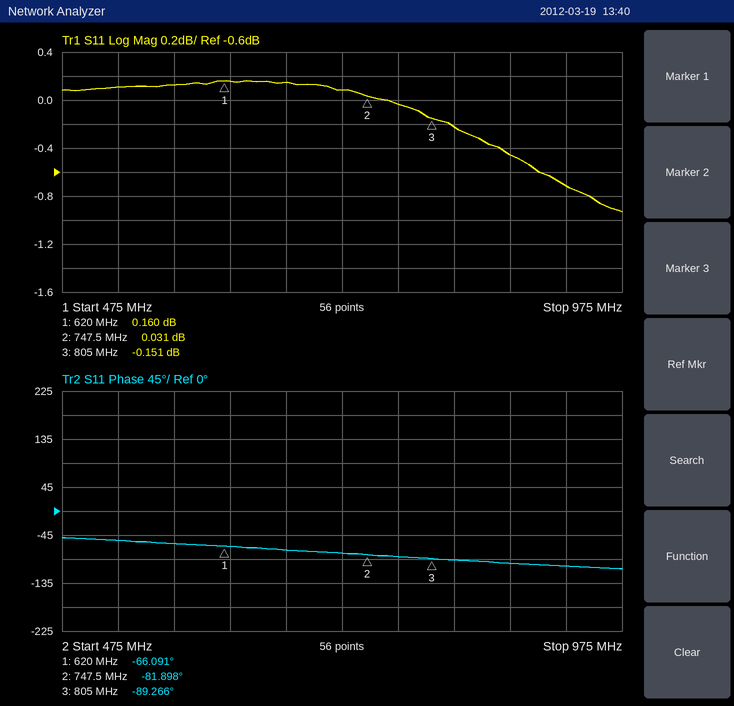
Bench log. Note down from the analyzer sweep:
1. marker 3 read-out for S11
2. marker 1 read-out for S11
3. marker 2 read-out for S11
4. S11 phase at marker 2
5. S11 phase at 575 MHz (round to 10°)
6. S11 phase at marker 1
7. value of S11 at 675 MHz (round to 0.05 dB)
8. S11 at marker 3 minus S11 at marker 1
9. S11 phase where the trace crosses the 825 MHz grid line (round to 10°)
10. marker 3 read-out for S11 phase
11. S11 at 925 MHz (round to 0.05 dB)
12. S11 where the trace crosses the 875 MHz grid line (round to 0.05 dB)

-0.151 dB
0.160 dB
0.031 dB
-81.898°
-60°
-66.091°
0.15 dB
-0.311 dB
-90°
-89.266°
-0.70 dB
-0.45 dB
